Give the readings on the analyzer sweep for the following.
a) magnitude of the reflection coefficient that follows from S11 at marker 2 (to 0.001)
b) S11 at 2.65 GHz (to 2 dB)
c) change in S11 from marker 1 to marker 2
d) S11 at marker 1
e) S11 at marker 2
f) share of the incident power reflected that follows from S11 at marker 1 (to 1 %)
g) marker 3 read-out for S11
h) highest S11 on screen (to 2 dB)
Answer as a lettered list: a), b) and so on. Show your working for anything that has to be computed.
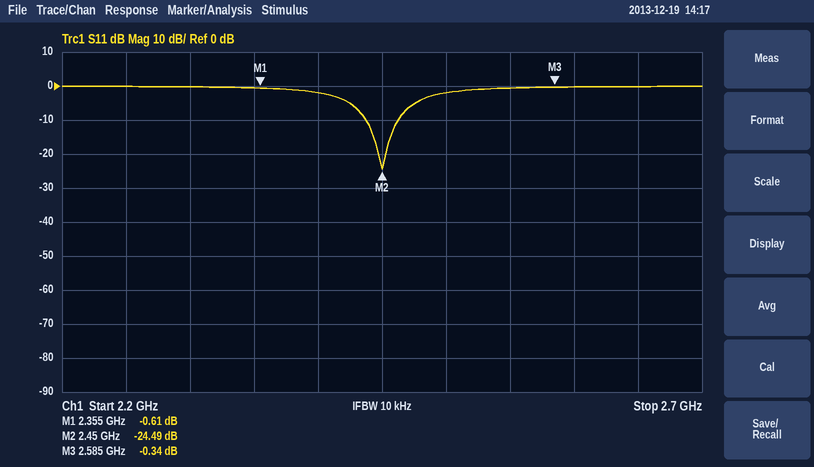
a) 10^(-24.49/20) ≈ 0.060
b) 0 dB
c) -24.49 − (-0.61) = -23.88 dB
d) -0.61 dB
e) -24.49 dB
f) 10^(-0.61/10) ≈ 87 %
g) -0.34 dB
h) 0 dB
